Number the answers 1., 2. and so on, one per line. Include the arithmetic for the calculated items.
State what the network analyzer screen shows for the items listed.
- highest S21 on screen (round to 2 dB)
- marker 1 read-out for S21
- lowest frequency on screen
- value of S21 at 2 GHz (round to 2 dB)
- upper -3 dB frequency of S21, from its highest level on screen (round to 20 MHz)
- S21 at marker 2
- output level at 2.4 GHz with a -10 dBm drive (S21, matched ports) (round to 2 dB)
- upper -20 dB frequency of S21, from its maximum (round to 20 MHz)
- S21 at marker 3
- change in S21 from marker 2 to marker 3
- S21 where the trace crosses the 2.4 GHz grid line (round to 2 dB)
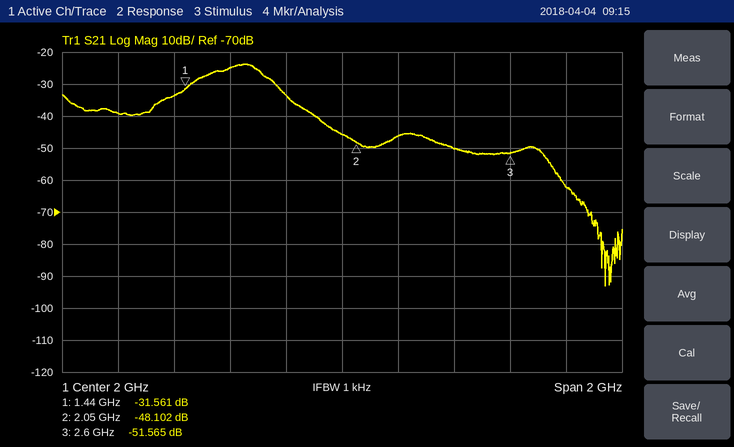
1. -24 dB
2. -31.561 dB
3. 1 GHz
4. -46 dB
5. 1.72 GHz
6. -48.102 dB
7. -10 dBm + (-50 dB) = -60 dBm
8. 1.96 GHz
9. -51.565 dB
10. -51.565 − (-48.102) = -3.463 dB
11. -50 dB
